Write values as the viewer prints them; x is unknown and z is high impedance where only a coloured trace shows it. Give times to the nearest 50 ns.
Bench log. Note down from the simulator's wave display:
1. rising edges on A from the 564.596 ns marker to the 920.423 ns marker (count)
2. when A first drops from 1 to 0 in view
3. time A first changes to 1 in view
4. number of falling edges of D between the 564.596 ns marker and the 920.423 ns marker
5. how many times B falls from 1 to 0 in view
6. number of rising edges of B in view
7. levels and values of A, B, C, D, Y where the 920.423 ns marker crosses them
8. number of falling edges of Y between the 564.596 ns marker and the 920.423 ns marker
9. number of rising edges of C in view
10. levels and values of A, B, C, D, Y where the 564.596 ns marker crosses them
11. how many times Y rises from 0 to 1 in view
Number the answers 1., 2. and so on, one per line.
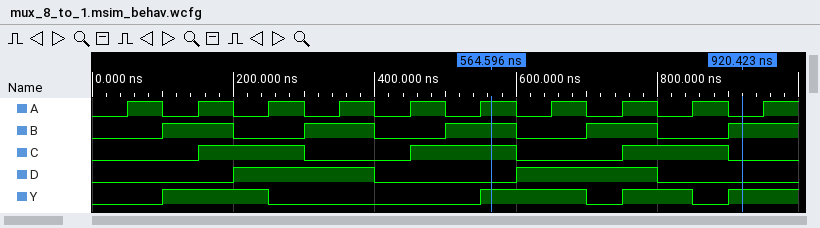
1. 3
2. 100 ns
3. 50 ns
4. 1
5. 4
6. 5
7. A=0, B=1, C=0, D=0, Y=1
8. 2
9. 3
10. A=1, B=1, C=1, D=0, Y=1
11. 4
